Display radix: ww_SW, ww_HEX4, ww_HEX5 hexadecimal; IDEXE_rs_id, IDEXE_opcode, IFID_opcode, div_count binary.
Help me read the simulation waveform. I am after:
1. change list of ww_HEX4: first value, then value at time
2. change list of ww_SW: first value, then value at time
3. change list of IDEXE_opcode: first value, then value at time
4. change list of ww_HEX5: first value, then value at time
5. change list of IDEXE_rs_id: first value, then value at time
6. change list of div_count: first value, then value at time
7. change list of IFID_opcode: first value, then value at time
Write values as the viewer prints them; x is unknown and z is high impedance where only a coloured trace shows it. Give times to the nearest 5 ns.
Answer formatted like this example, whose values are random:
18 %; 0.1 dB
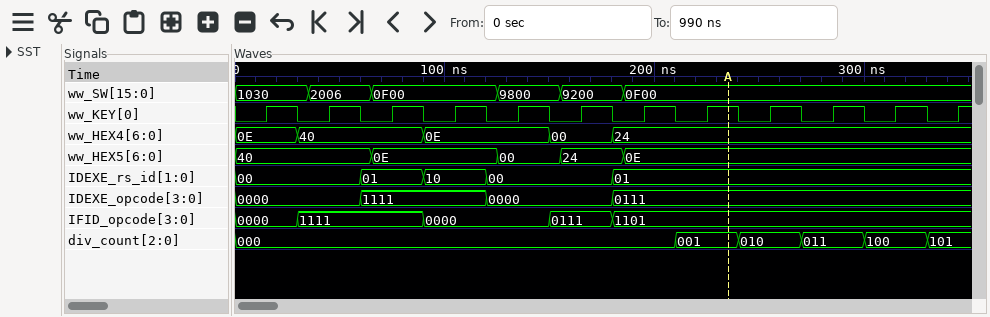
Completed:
0E, 40 at 30 ns, 0E at 90 ns, 00 at 150 ns, 24 at 180 ns; 1030, 2006 at 35 ns, 0F00 at 65 ns, 9800 at 125 ns, 9200 at 155 ns, 0F00 at 185 ns; 0000, 1111 at 60 ns, 0000 at 120 ns, 0111 at 180 ns; 40, 0E at 65 ns, 00 at 125 ns, 24 at 155 ns, 0E at 185 ns; 00, 01 at 60 ns, 10 at 90 ns, 00 at 120 ns, 01 at 180 ns; 000, 001 at 210 ns, 010 at 240 ns, 011 at 270 ns, 100 at 300 ns, 101 at 330 ns; 0000, 1111 at 30 ns, 0000 at 90 ns, 0111 at 150 ns, 1101 at 180 ns
